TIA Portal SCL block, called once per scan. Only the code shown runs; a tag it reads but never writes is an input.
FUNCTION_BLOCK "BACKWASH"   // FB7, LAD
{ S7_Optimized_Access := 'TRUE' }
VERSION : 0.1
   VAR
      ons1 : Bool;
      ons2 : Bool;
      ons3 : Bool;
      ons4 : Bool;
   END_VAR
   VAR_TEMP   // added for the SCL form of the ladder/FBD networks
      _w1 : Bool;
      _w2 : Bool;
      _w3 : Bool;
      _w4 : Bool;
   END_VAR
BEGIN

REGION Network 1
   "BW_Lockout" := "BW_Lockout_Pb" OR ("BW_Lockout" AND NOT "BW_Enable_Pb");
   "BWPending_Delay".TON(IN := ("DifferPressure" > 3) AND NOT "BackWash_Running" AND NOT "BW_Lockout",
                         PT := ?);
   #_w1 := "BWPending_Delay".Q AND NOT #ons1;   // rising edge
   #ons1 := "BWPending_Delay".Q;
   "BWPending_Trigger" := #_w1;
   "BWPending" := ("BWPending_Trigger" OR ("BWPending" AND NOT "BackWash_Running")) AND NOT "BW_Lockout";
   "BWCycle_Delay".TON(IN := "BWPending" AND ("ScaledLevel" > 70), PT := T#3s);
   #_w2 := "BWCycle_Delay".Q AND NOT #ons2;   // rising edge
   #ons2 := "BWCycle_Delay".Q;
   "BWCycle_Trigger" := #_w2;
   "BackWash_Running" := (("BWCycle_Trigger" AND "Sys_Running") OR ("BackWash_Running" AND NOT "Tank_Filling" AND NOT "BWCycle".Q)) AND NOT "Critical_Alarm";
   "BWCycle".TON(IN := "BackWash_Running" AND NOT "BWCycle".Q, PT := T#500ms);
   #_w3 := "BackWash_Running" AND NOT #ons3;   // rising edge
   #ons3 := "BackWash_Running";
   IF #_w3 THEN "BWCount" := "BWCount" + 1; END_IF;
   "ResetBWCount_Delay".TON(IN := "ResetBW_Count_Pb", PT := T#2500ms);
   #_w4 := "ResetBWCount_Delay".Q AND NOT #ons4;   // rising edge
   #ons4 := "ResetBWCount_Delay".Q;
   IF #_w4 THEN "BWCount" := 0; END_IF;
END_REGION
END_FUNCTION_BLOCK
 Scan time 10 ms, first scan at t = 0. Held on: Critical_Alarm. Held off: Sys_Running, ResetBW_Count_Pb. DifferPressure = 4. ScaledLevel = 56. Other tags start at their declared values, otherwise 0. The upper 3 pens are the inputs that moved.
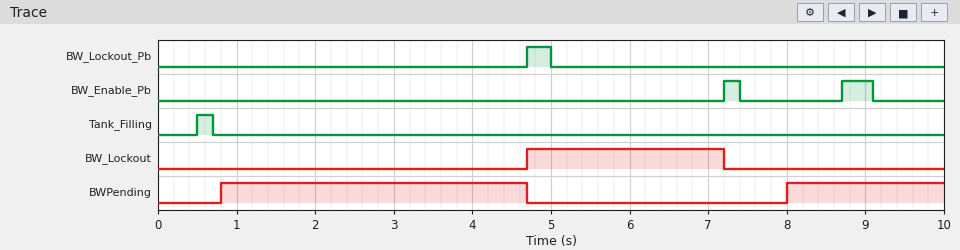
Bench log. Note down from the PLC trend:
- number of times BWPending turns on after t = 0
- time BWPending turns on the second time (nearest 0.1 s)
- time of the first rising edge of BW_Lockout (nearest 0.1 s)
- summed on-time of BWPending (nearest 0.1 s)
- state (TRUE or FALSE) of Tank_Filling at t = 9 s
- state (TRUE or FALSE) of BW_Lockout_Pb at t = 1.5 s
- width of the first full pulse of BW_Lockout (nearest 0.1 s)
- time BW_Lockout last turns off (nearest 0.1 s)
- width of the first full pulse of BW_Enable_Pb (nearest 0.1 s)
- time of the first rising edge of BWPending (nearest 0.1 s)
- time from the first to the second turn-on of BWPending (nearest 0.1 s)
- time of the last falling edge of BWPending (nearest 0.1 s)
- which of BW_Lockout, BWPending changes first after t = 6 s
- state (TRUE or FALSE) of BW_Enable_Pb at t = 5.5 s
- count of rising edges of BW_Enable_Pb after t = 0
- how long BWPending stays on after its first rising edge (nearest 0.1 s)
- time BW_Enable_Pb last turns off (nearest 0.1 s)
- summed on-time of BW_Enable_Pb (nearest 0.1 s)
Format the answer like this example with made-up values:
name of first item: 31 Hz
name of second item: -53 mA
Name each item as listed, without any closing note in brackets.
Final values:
number of times BWPending turns on after t = 0: 2
time BWPending turns on the second time: 8.0 s
time of the first rising edge of BW_Lockout: 4.7 s
summed on-time of BWPending: 5.9 s
state (TRUE or FALSE) of Tank_Filling at t = 9 s: FALSE
state (TRUE or FALSE) of BW_Lockout_Pb at t = 1.5 s: FALSE
width of the first full pulse of BW_Lockout: 2.5 s
time BW_Lockout last turns off: 7.2 s
width of the first full pulse of BW_Enable_Pb: 0.2 s
time of the first rising edge of BWPending: 0.8 s
time from the first to the second turn-on of BWPending: 7.2 s
time of the last falling edge of BWPending: 4.7 s
which of BW_Lockout, BWPending changes first after t = 6 s: BW_Lockout
state (TRUE or FALSE) of BW_Enable_Pb at t = 5.5 s: FALSE
count of rising edges of BW_Enable_Pb after t = 0: 2
how long BWPending stays on after its first rising edge: 3.9 s
time BW_Enable_Pb last turns off: 9.1 s
summed on-time of BW_Enable_Pb: 0.6 s
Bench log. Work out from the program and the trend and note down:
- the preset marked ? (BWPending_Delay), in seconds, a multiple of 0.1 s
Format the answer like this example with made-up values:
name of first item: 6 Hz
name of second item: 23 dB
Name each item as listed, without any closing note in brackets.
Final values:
the preset marked ? (BWPending_Delay), in seconds, a multiple of 0.1 s: 0.8 s
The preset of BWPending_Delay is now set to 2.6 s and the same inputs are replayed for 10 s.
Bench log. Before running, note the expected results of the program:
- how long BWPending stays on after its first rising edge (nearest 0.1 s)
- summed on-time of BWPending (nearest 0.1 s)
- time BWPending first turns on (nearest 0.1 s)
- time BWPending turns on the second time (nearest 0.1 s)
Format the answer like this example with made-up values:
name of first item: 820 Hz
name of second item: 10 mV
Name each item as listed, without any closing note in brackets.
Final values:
how long BWPending stays on after its first rising edge: 2.1 s
summed on-time of BWPending: 2.3 s
time BWPending first turns on: 2.6 s
time BWPending turns on the second time: 9.8 s
